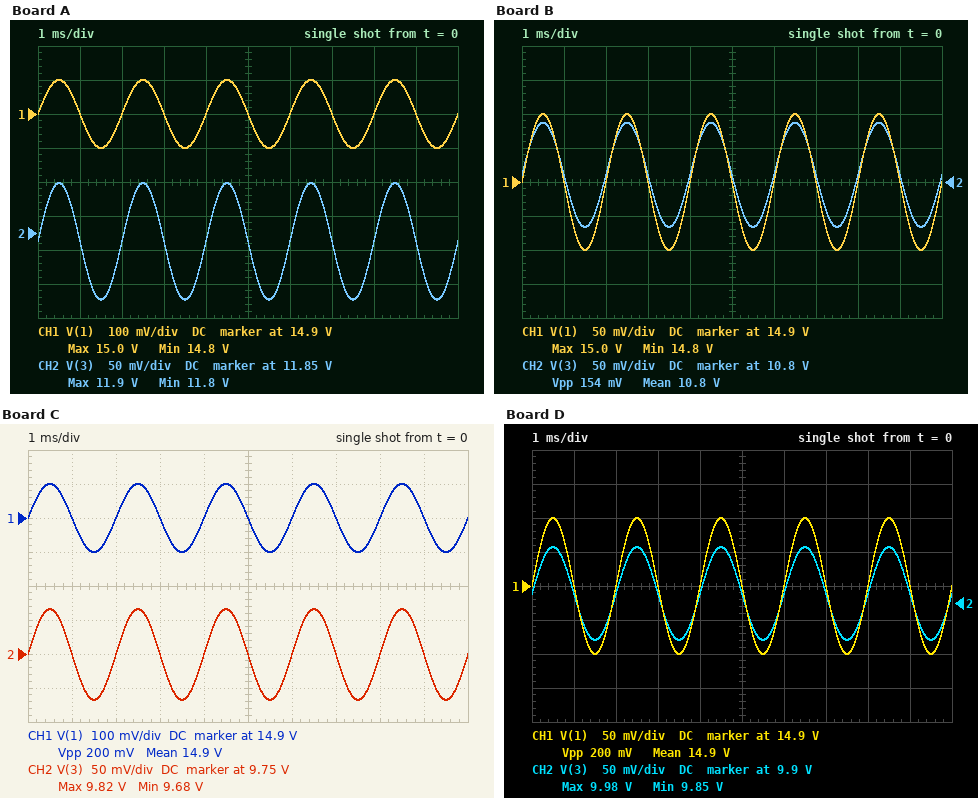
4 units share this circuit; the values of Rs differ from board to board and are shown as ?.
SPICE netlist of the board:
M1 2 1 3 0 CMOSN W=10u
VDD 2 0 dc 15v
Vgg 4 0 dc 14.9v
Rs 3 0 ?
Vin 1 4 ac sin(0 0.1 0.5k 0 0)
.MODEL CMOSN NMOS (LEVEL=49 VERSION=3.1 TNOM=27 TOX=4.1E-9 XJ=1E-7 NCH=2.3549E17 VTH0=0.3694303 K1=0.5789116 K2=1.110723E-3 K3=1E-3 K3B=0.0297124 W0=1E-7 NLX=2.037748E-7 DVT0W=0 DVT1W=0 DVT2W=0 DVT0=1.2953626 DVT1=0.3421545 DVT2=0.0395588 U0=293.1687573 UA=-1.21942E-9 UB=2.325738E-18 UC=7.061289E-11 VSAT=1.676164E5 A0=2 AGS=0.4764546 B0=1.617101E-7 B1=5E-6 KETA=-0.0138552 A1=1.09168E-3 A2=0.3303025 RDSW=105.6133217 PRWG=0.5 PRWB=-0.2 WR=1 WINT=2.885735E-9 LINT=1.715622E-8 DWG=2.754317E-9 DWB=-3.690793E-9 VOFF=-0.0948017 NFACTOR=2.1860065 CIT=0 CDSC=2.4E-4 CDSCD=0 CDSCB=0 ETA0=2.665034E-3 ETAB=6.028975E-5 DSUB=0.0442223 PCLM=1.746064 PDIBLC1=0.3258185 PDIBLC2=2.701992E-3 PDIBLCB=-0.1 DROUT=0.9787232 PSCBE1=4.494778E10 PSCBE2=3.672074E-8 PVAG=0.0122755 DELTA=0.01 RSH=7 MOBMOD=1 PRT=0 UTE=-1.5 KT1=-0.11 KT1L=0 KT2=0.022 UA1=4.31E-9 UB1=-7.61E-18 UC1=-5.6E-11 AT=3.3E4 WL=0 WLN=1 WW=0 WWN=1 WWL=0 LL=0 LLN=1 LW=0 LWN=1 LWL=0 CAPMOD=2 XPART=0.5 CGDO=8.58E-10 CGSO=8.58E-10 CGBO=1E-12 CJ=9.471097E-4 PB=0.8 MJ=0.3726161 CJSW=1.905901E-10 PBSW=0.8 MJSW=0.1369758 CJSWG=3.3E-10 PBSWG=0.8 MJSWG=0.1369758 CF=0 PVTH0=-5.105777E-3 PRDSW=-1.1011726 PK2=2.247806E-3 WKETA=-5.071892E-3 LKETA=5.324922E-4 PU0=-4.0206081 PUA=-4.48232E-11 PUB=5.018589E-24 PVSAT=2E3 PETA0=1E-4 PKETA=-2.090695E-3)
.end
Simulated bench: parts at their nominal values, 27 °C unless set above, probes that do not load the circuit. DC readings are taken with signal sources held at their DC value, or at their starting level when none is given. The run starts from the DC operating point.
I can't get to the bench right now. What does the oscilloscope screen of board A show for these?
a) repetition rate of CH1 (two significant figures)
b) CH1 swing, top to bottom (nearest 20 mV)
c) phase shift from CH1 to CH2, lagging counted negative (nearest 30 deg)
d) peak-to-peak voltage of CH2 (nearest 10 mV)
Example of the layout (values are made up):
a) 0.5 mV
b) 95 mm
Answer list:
a) 500 Hz
b) 200 mV
c) 0 deg
d) 170 mV
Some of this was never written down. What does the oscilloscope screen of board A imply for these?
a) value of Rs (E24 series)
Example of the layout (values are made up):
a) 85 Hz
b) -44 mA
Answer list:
a) 62 kΩ
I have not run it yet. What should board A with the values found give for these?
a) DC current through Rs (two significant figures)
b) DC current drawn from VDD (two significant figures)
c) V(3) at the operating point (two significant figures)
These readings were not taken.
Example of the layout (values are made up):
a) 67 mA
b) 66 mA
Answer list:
a) 190 µA
b) 190 µA
c) 12 V
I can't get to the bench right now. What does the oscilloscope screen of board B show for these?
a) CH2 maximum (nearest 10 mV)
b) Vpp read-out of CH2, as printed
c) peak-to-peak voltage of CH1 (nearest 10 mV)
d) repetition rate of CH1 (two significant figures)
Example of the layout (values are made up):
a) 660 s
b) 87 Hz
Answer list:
a) 10.89 V
b) 154 mV
c) 200 mV
d) 500 Hz
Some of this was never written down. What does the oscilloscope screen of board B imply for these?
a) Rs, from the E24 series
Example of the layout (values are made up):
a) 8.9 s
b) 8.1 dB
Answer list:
a) 22 kΩ
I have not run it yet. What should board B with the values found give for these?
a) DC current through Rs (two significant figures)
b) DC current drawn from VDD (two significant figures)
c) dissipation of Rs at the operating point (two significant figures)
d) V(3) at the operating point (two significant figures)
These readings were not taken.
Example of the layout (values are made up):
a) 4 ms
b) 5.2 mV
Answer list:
a) 490 µA
b) 490 µA
c) 5.3 mW
d) 11 V
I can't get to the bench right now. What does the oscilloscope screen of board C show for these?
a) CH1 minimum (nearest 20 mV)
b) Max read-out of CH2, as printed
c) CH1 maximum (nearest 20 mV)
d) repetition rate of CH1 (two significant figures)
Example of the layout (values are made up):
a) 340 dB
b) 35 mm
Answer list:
a) 14.80 V
b) 9.82 V
c) 15.00 V
d) 500 Hz
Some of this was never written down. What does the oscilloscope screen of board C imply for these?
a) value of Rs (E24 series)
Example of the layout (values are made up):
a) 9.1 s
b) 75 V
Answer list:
a) 12 kΩ
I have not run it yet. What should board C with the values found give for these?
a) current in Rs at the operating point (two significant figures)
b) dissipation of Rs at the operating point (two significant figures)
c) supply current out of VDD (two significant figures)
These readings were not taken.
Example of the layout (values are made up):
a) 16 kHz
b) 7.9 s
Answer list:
a) 810 µA
b) 7.9 mW
c) 810 µA
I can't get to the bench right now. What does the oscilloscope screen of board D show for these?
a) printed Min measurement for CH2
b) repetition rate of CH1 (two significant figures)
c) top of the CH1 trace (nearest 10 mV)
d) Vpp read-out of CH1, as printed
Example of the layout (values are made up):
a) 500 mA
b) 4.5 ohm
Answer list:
a) 9.85 V
b) 500 Hz
c) 15.00 V
d) 200 mV
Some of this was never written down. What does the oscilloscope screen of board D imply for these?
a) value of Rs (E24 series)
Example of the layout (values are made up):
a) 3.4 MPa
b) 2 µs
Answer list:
a) 13 kΩ
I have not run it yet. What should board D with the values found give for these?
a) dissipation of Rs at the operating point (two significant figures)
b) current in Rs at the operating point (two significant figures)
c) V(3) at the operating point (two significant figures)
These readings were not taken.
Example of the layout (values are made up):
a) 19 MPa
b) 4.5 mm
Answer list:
a) 7.6 mW
b) 760 µA
c) 9.9 V
